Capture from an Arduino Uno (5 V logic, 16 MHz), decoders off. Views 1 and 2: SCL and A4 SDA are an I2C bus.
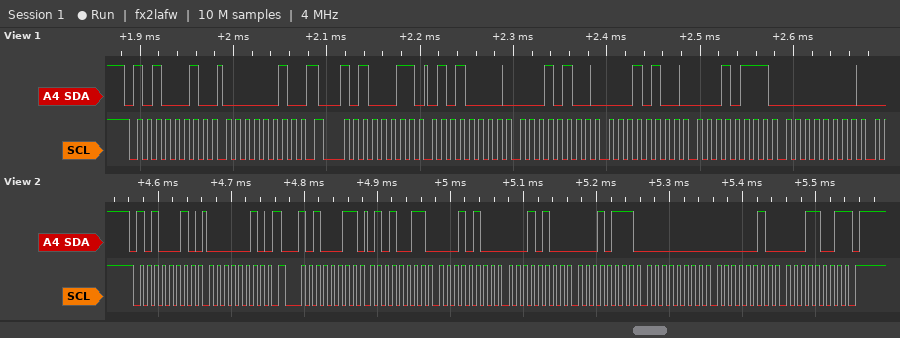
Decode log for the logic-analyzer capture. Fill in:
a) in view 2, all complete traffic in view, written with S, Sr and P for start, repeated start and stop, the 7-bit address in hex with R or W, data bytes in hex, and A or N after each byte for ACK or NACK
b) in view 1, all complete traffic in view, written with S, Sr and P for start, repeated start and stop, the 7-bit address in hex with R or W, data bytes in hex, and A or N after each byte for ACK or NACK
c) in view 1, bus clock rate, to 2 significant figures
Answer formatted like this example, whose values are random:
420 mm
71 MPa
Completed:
S 51W A 02 A Sr 51R A 53 A 14 A 14 A 17 A 00 A 02 A 19 N P
S 51W A 02 A Sr 51R A 50 A 14 A 14 A 17 A 00 A
100 kHz
